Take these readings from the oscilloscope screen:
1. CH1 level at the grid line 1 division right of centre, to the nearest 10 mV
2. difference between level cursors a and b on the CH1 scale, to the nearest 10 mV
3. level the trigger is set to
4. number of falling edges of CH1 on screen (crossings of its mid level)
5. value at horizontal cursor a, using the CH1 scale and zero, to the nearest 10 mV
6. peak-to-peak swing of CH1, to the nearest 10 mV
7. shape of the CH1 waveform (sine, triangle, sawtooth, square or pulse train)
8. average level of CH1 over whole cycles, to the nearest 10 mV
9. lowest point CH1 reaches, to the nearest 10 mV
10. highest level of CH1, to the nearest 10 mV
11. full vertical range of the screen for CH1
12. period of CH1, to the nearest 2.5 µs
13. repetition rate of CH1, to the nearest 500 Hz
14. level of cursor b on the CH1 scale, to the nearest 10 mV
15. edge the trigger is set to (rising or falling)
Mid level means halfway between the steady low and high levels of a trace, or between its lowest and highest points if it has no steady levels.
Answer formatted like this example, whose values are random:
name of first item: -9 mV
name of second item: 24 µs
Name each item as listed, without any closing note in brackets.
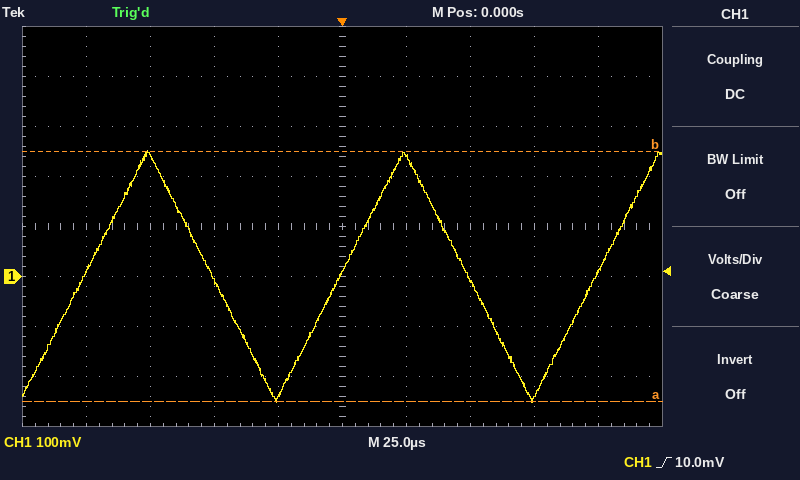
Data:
CH1 level at the grid line 1 division right of centre, to the nearest 10 mV: 240 mV
difference between level cursors a and b on the CH1 scale, to the nearest 10 mV: 500 mV
level the trigger is set to: 10.0 mV
number of falling edges of CH1 on screen: 2
value at horizontal cursor a, using the CH1 scale and zero, to the nearest 10 mV: -250 mV
peak-to-peak swing of CH1, to the nearest 10 mV: 500 mV
shape of the CH1 waveform: triangle
average level of CH1 over whole cycles, to the nearest 10 mV: 0 mV
lowest point CH1 reaches, to the nearest 10 mV: -250 mV
highest level of CH1, to the nearest 10 mV: 250 mV
full vertical range of the screen for CH1: 800 mV
period of CH1, to the nearest 2.5 µs: 100.0 µs
repetition rate of CH1, to the nearest 500 Hz: 10.0 kHz
level of cursor b on the CH1 scale, to the nearest 10 mV: 250 mV
edge the trigger is set to: rising
